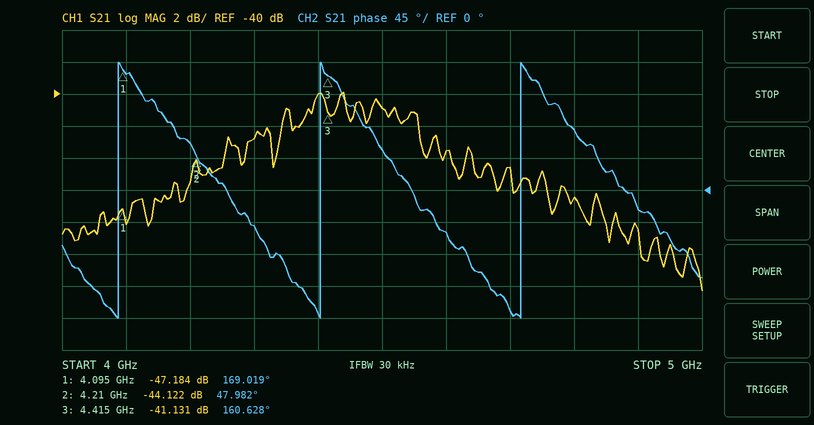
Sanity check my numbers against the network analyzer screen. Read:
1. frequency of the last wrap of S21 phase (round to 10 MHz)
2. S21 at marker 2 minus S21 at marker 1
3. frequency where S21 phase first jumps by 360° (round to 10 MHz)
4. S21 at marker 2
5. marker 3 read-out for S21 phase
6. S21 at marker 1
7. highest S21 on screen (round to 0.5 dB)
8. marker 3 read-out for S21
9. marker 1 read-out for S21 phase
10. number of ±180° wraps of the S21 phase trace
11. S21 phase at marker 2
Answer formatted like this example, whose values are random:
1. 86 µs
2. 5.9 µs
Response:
1. 4.72 GHz
2. 3.062 dB
3. 4.09 GHz
4. -44.122 dB
5. 160.628°
6. -47.184 dB
7. -40.0 dB
8. -41.131 dB
9. 169.019°
10. 3
11. 47.982°
